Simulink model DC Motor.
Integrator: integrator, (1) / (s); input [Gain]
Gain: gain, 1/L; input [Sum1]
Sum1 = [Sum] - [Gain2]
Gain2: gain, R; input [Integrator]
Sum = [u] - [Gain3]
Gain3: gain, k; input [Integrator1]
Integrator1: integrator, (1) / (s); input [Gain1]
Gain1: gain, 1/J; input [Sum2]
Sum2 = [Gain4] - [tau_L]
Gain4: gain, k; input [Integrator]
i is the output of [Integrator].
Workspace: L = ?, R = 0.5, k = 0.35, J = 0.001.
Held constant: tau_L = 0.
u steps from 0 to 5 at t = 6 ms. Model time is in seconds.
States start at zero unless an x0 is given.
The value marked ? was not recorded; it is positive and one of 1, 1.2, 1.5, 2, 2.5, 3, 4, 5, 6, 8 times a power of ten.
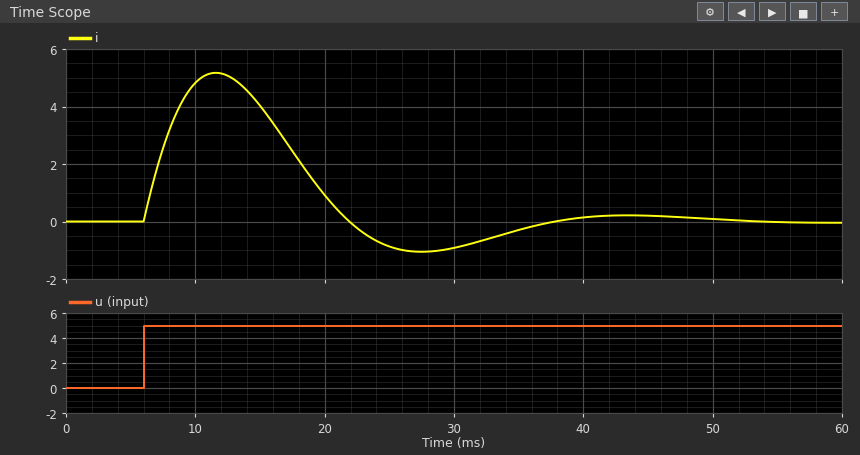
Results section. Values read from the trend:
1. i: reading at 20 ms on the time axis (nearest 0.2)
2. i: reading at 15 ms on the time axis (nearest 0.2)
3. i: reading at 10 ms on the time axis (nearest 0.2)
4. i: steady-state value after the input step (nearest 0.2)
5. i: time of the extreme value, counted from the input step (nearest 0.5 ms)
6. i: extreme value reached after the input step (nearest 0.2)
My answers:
1.0
4.0
4.8
0.0
5.5 ms
5.2
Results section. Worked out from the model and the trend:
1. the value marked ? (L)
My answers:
0.0025
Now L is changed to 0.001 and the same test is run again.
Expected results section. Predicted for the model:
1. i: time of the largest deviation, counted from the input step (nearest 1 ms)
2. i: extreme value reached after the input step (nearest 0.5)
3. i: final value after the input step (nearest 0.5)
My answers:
3 ms
6.5
0.0
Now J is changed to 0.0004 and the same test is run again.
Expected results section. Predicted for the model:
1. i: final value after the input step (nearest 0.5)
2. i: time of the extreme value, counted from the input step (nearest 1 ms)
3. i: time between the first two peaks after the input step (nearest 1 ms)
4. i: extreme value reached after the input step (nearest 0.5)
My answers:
0.0
4 ms
19 ms
4.0
